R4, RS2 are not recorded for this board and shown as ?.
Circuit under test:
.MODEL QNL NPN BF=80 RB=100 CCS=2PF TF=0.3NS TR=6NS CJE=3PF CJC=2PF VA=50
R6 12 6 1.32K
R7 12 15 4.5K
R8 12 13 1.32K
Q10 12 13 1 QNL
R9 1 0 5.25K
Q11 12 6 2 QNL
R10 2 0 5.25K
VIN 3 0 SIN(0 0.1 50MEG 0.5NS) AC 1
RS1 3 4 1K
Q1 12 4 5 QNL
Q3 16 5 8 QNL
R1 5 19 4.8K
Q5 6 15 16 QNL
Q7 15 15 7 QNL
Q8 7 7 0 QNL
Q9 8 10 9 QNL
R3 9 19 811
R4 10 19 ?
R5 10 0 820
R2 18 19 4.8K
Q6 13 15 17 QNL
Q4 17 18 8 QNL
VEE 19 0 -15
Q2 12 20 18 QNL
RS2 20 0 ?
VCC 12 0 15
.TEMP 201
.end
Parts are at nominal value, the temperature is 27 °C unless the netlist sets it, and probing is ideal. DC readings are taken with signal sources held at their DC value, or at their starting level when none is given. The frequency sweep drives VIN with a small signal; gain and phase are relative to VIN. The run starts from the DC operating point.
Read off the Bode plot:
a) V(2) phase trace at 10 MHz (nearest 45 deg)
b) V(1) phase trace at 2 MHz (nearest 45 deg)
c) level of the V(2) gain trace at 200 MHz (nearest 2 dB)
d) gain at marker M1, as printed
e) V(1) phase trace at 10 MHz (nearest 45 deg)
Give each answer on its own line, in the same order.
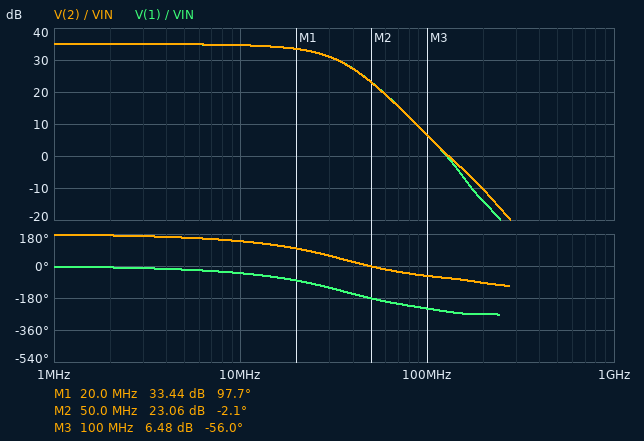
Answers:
135 deg
0 deg
-10 dB
33.44 dB
-45 deg
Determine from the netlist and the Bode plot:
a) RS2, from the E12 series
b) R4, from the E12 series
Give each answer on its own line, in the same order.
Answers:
820 Ω
820 Ω
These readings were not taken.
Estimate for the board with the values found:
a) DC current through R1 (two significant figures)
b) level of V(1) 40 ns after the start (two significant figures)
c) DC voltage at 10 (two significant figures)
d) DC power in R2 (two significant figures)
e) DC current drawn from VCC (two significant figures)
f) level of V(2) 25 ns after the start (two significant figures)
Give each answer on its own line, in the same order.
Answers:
3.0 mA
9.0 V
-7.5 V
43 mW
21 mA
11 V
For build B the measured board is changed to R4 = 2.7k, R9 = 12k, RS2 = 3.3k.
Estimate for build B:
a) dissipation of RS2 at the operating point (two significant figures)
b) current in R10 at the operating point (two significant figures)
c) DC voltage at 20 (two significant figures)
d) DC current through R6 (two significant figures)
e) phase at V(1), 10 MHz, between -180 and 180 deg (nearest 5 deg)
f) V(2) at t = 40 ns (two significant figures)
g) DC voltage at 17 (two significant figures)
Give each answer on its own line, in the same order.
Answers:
2.7 µW
230 µA
-95 mV
10 mA
-45 deg
1.2 V
580 mV
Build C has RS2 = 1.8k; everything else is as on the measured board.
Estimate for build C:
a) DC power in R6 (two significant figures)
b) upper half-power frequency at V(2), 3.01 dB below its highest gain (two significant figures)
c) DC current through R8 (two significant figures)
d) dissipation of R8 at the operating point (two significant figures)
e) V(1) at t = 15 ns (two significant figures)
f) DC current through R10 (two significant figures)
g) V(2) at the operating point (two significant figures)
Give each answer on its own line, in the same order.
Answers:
34 mW
26 MHz
3.1 mA
13 mW
12 V
1.5 mA
7.8 V
